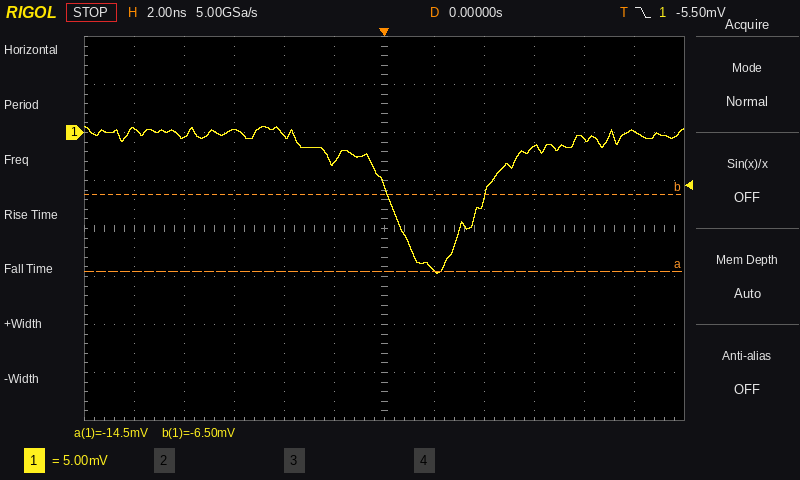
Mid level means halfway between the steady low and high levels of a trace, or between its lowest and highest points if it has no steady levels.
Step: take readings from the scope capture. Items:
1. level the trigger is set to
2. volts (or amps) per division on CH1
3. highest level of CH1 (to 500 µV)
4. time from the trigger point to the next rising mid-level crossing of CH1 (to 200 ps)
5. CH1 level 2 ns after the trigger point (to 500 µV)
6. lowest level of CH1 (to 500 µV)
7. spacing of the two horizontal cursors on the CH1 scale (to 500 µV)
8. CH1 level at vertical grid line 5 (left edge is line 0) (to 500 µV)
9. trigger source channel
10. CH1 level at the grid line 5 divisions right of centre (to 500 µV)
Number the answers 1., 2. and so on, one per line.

1. -5.50 mV
2. 5 mV
3. 500 µV
4. 4.0 ns
5. -14.5 mV
6. -14.5 mV
7. 8.0 mV
8. -3.0 mV
9. CH1
10. 0.0 mV
